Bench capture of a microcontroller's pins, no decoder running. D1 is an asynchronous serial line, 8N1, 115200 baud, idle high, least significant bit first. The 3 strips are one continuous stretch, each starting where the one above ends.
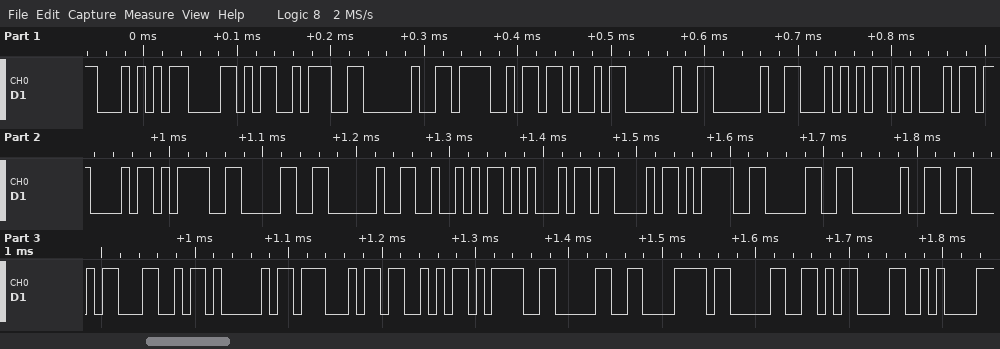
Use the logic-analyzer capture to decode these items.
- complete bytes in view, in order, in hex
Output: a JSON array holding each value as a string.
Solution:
["54 58 3A 20 4F 4B 20 20 54 45 43 3D 30 20 52 45 43 3D 30 20 46 4C 41 47 53 3D 30 78 30 0D 0A"]
